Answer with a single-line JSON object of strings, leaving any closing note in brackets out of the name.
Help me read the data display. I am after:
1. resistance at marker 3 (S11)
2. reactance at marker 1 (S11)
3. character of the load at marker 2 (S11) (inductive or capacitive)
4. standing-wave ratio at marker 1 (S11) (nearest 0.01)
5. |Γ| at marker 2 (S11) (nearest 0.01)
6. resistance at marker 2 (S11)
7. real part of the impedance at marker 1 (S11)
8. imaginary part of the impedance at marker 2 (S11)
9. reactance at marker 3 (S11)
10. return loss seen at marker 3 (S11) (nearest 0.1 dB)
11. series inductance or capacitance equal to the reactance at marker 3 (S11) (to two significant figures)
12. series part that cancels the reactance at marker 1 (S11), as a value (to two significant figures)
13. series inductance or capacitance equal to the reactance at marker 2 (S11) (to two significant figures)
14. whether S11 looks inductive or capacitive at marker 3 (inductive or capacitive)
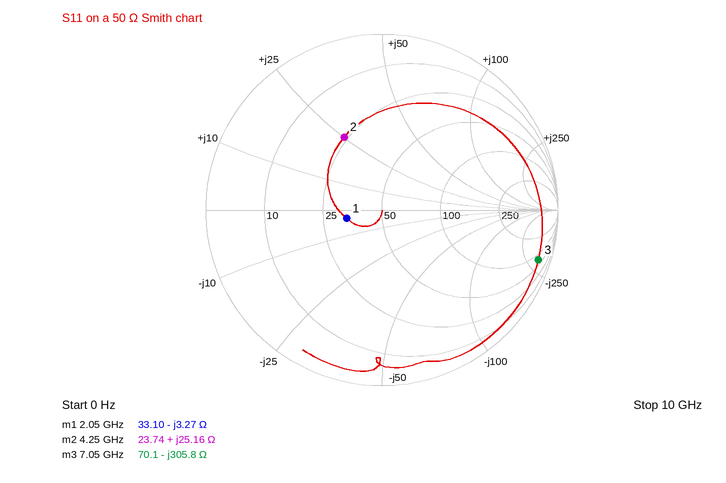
{"resistance at marker 3": "70.1 Ω", "reactance at marker 1": "-3.27 Ω", "character of the load at marker 2 (S11)": "inductive", "standing-wave ratio at marker 1 (S11)": "1.52", "|Γ| at marker 2 (S11)": "0.47", "resistance at marker 2": "23.74 Ω", "real part of the impedance at marker 1": "33.10 Ω", "imaginary part of the impedance at marker 2": "+25.16 Ω", "reactance at marker 3": "-305.8 Ω", "return loss seen at marker 3 (S11)": "0.6 dB", "series inductance or capacitance equal to the reactance at marker 3 (S11)": "74 fF", "series part that cancels the reactance at marker 1 (S11), as a value": "250 pH", "series inductance or capacitance equal to the reactance at marker 2 (S11)": "940 pH", "whether S11 looks inductive or capacitive at marker 3": "capacitive"}
